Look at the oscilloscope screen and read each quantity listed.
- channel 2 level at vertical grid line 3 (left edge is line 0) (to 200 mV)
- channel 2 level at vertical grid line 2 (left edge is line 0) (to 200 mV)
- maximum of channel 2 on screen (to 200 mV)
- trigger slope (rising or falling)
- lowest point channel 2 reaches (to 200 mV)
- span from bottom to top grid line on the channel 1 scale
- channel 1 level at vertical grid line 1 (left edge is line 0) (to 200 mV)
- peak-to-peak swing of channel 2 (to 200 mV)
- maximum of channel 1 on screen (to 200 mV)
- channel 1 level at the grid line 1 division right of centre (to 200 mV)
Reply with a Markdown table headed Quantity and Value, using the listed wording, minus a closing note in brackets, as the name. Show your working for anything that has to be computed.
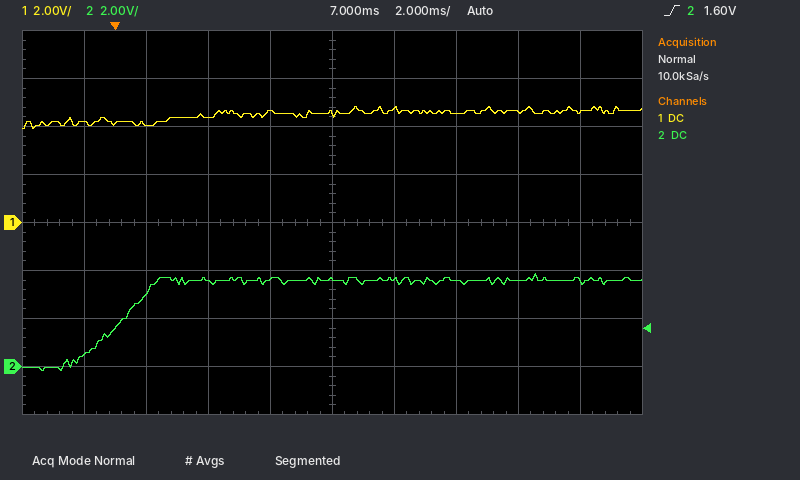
| Quantity | Value |
|---|---|
| channel 2 level at vertical grid line 3 (left edge is line 0) | 3.6 V |
| channel 2 level at vertical grid line 2 (left edge is line 0) | 3.0 V |
| maximum of channel 2 on screen | 3.8 V |
| trigger slope | rising |
| lowest point channel 2 reaches | -200 mV |
| span from bottom to top grid line on the channel 1 scale | 16 V |
| channel 1 level at vertical grid line 1 (left edge is line 0) | 4.2 V |
| peak-to-peak swing of channel 2 | 3.8 V − (-200 mV) = 4.0 V |
| maximum of channel 1 on screen | 4.8 V |
| channel 1 level at the grid line 1 division right of centre | 4.8 V |
